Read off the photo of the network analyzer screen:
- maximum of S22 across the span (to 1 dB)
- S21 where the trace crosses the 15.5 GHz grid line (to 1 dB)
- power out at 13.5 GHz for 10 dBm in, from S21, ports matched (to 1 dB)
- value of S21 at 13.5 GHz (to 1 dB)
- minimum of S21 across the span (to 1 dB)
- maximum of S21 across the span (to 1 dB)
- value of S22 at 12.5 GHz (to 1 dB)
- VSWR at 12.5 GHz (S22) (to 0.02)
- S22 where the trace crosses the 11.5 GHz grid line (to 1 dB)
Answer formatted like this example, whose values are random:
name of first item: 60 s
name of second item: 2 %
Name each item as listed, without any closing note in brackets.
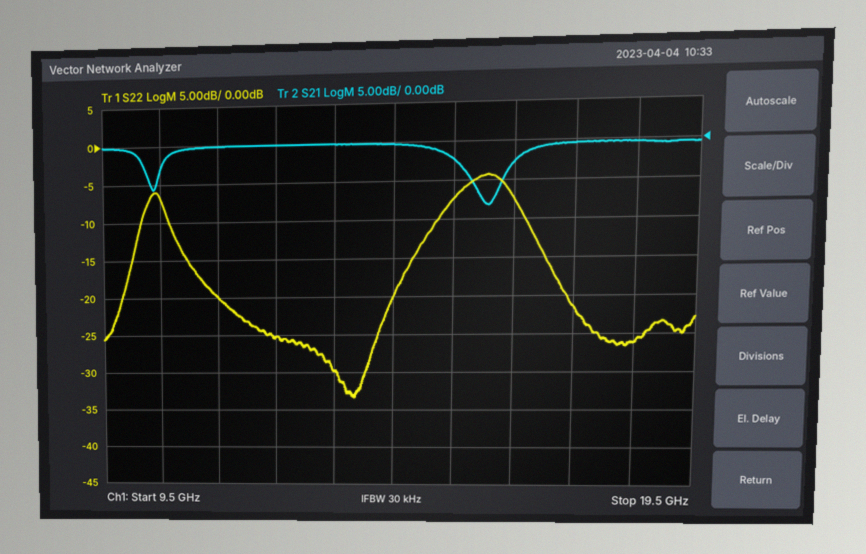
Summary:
maximum of S22 across the span: -4 dB
S21 where the trace crosses the 15.5 GHz grid line: -2 dB
power out at 13.5 GHz for 10 dBm in, from S21, ports matched: 10 dBm
value of S21 at 13.5 GHz: 0 dB
minimum of S21 across the span: -8 dB
maximum of S21 across the span: 0 dB
value of S22 at 12.5 GHz: -25 dB
VSWR at 12.5 GHz (S22): 1.12
S22 where the trace crosses the 11.5 GHz grid line: -20 dB
